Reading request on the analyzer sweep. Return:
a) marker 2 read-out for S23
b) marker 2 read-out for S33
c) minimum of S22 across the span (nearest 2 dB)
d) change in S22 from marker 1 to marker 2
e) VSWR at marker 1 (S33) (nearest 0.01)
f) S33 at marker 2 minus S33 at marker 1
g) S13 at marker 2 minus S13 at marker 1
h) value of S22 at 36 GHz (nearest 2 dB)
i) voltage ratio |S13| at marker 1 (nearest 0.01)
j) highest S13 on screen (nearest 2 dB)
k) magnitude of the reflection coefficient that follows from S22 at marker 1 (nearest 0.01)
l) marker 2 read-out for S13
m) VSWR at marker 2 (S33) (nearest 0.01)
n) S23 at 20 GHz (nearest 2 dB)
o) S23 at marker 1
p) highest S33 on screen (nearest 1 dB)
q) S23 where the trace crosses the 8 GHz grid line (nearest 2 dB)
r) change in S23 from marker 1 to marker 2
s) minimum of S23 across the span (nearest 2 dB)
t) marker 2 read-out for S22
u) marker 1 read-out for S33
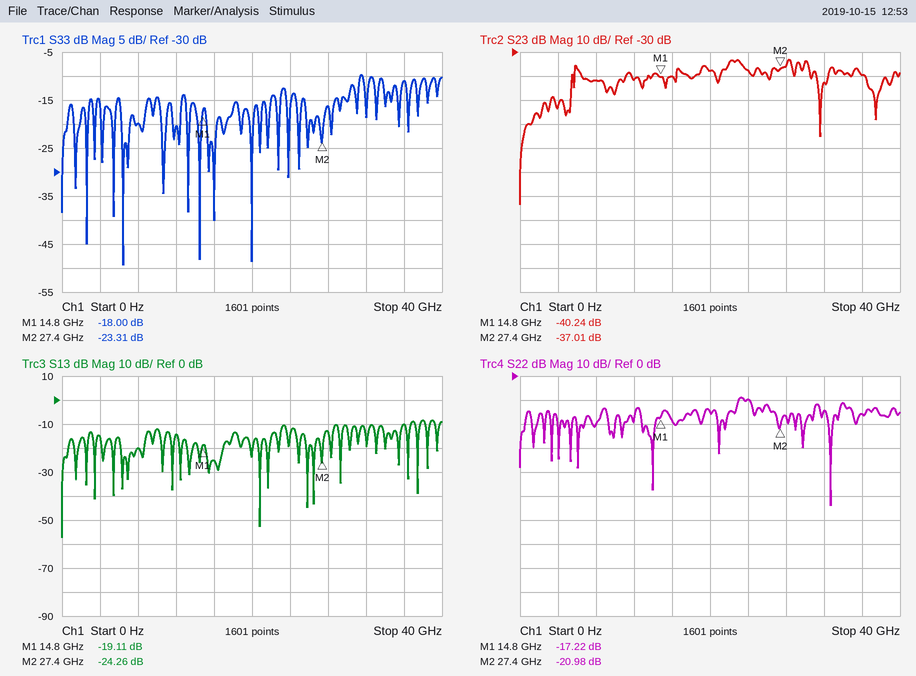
-37.01 dB
-23.31 dB
-54 dB
-3.76 dB
1.29
-5.31 dB
-5.15 dB
-16 dB
0.11
-8 dB
0.14
-24.26 dB
1.15
-38 dB
-40.24 dB
-10 dB
-42 dB
3.23 dB
-94 dB
-20.98 dB
-18.00 dB
